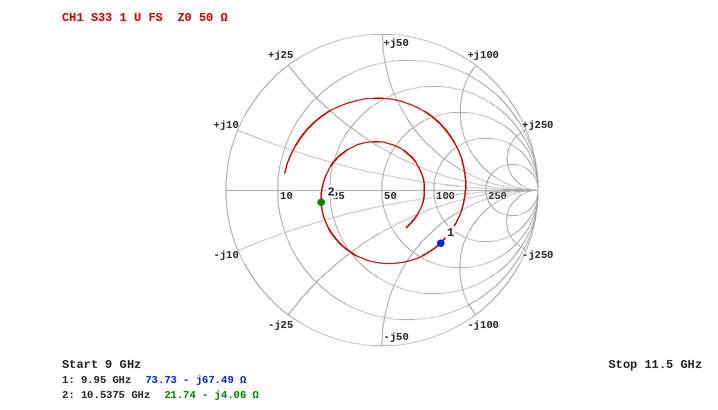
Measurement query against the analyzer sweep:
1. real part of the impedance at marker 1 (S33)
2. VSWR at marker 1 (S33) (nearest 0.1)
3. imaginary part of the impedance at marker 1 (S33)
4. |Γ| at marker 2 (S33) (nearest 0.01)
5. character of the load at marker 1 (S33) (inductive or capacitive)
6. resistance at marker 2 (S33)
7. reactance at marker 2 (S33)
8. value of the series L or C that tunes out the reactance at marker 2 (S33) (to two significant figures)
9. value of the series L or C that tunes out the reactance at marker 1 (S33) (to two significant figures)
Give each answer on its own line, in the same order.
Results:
73.73 Ω
3.1
-67.49 Ω
0.40
capacitive
21.74 Ω
-4.06 Ω
61 pH
1.1 nH
